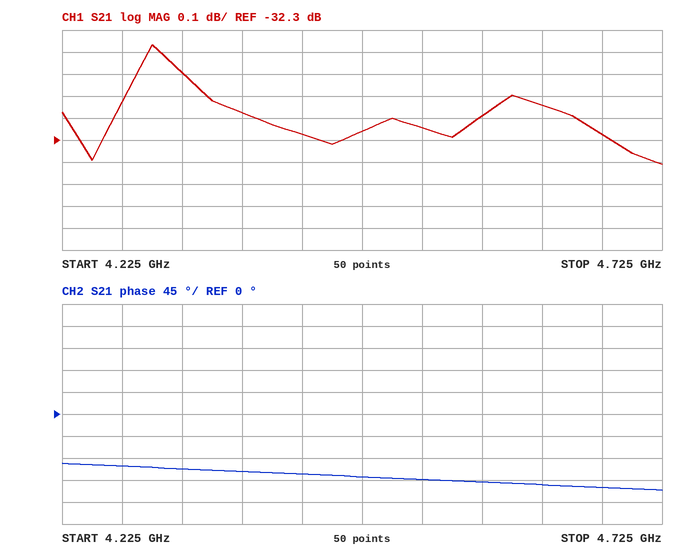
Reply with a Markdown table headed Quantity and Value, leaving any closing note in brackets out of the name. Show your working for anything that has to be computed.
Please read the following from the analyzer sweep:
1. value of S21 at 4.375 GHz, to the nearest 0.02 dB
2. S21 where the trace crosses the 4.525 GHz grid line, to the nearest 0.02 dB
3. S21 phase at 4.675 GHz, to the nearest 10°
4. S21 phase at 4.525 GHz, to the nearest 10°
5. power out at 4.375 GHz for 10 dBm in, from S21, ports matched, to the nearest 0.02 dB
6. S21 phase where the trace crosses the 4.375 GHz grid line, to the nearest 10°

| Quantity | Value |
|---|---|
| value of S21 at 4.375 GHz, to the nearest 0.02 dB | -32.18 dB |
| S21 where the trace crosses the 4.525 GHz grid line, to the nearest 0.02 dB | -32.24 dB |
| S21 phase at 4.675 GHz, to the nearest 10° | -150° |
| S21 phase at 4.525 GHz, to the nearest 10° | -130° |
| power out at 4.375 GHz for 10 dBm in, from S21, ports matched, to the nearest 0.02 dB | 10 dBm + (-32.18 dB) = -22.18 dBm |
| S21 phase where the trace crosses the 4.375 GHz grid line, to the nearest 10° | -120° |
